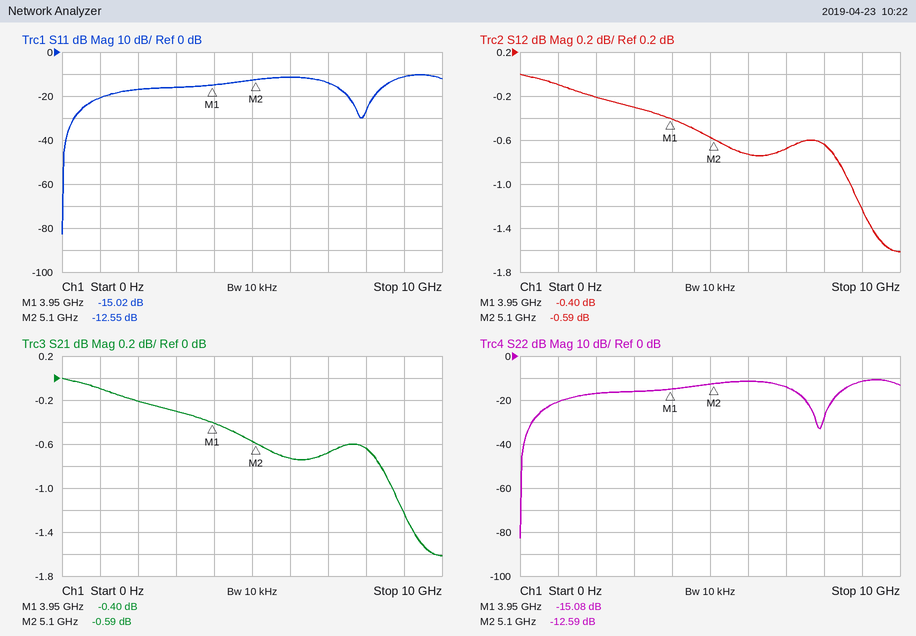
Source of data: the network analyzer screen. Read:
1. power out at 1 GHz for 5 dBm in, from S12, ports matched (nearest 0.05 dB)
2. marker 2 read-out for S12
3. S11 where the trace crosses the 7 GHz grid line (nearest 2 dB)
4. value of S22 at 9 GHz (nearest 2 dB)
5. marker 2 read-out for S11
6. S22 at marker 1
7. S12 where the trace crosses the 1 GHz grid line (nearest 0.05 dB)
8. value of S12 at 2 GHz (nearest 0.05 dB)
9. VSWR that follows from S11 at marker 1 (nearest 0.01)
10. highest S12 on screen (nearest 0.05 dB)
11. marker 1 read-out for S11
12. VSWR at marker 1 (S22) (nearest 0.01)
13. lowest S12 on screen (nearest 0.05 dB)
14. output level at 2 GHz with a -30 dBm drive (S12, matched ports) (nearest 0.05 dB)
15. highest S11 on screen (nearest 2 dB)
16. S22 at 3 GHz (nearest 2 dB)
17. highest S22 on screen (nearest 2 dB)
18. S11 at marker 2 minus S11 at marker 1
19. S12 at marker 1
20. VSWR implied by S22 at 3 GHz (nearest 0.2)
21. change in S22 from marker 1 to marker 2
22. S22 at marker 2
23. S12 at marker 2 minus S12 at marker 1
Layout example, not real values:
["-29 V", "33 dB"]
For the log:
["4.90 dBm", "-0.59 dB", "-14 dB", "-12 dB", "-12.55 dB", "-15.08 dB", "-0.10 dB", "-0.20 dB", "1.43", "0.00 dB", "-15.02 dB", "1.43", "-1.60 dB", "-30.20 dBm", "-10 dB", "-16 dB", "-10 dB", "2.47 dB", "-0.40 dB", "1.4", "2.49 dB", "-12.59 dB", "-0.19 dB"]
